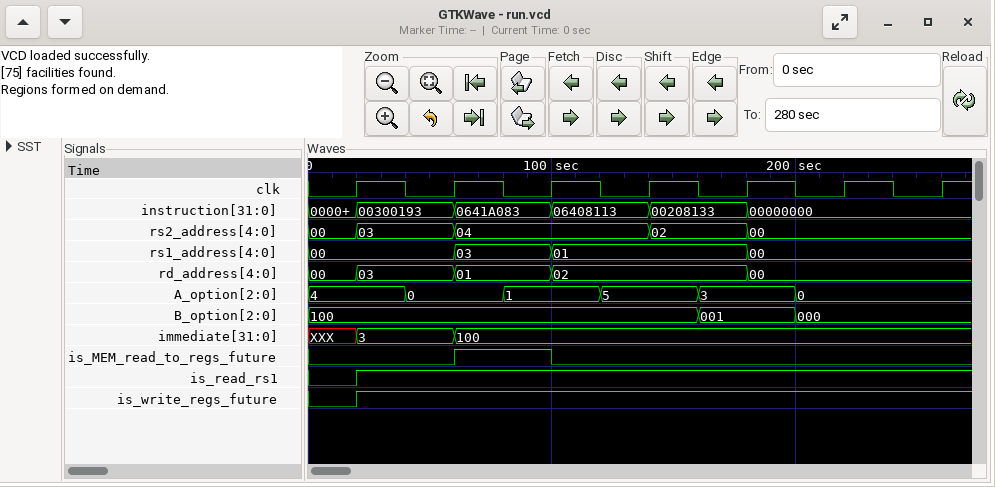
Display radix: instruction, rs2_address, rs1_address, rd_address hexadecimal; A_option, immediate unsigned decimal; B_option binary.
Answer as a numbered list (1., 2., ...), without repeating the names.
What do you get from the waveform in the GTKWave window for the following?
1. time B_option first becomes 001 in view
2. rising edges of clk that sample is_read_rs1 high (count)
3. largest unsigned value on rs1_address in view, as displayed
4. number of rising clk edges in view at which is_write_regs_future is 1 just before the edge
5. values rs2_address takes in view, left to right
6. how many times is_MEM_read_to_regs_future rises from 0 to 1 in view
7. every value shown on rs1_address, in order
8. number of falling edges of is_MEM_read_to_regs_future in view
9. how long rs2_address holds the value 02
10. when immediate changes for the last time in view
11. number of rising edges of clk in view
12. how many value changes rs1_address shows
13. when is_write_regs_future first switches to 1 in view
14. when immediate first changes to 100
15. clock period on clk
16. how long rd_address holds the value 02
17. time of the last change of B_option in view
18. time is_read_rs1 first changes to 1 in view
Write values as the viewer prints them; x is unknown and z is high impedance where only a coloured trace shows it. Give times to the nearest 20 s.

1. 160 s
2. 6
3. 03
4. 6
5. 00, 03, 04, 02, 00
6. 1
7. 00, 03, 01, 00
8. 1
9. 40 s
10. 60 s
11. 7
12. 3
13. 20 s
14. 60 s
15. 40 s
16. 80 s
17. 200 s
18. 20 s
